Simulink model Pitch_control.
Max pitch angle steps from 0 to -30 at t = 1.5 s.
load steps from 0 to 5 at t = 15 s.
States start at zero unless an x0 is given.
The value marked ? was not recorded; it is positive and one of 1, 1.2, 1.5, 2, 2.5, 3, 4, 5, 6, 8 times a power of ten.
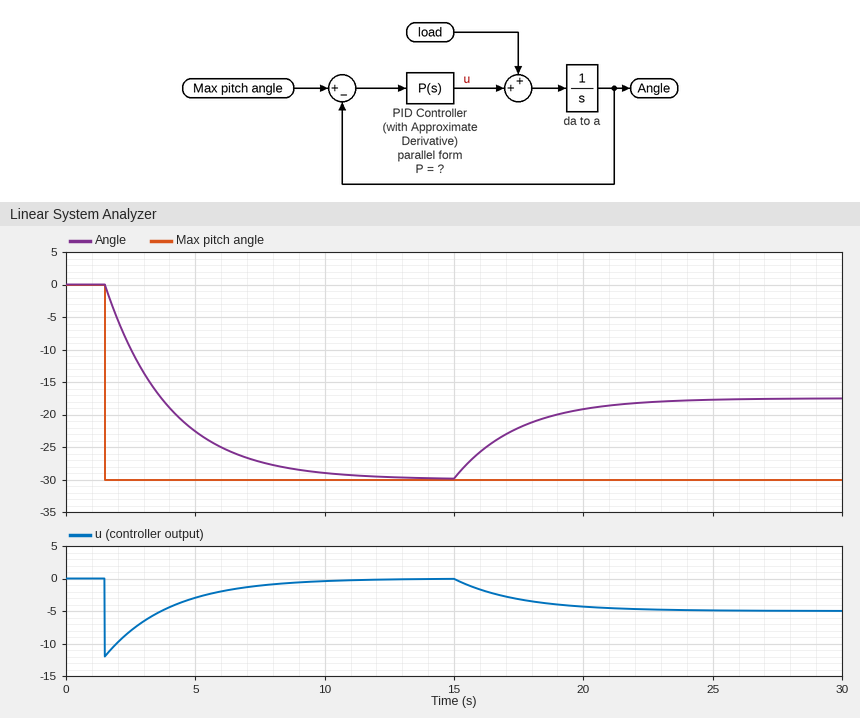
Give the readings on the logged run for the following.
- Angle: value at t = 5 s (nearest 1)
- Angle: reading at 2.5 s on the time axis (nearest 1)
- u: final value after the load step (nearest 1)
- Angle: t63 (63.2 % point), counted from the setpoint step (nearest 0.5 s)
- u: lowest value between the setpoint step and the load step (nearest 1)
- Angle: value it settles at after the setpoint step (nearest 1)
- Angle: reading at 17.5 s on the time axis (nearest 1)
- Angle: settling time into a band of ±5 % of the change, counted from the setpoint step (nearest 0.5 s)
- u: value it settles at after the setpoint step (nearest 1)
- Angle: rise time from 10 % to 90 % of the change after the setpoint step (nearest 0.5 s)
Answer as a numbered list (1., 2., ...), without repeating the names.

1. -23
2. -10
3. -5
4. 2.5 s
5. -12
6. -30
7. -22
8. 7.5 s
9. 0
10. 5.5 s
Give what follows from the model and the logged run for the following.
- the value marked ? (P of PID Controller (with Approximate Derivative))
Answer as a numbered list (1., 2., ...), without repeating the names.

1. 0.4
